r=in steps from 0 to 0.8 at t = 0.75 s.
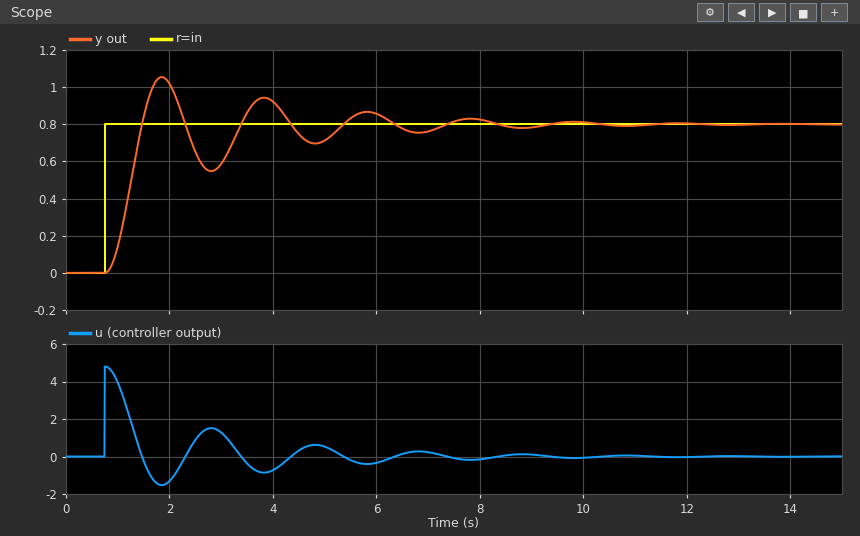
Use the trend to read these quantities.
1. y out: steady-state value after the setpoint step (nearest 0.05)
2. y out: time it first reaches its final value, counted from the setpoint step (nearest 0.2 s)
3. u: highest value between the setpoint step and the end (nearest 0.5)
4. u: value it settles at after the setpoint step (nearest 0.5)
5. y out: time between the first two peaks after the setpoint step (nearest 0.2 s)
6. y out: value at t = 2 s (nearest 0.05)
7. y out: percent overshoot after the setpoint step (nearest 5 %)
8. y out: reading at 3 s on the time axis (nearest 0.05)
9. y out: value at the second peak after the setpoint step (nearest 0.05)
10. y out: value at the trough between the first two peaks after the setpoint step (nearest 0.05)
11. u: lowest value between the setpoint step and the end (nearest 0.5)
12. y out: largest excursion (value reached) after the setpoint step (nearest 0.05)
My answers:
0.80
0.8 s
5.0
0.0
2.0 s
1.00
30 %
0.60
0.95
0.55
-1.5
1.05
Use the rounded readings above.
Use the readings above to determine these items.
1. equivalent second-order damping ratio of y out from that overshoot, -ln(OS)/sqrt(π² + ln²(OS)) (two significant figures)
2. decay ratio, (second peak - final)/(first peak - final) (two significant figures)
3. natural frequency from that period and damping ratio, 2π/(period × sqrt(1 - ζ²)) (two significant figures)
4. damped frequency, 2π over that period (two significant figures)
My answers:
0.36
0.60
3.4 rad/s
3.1 rad/s
